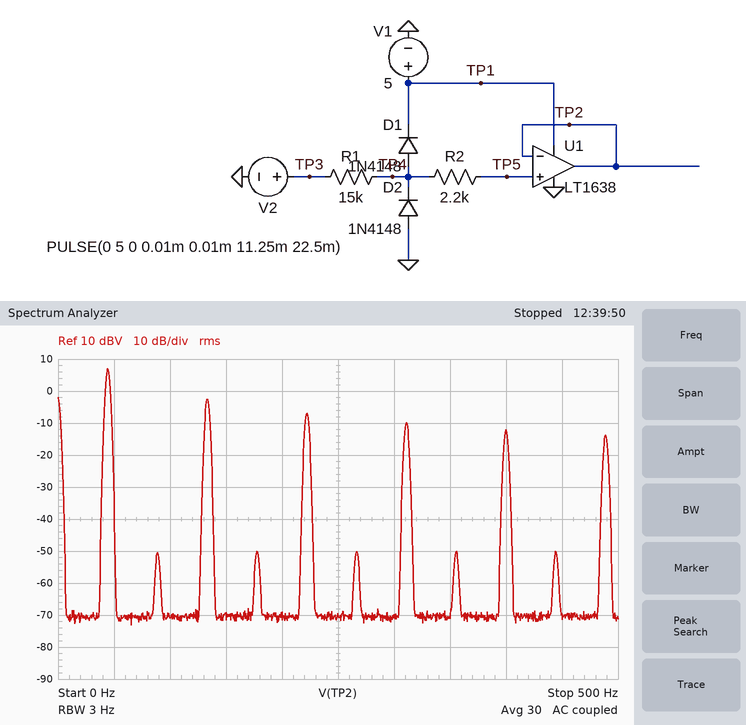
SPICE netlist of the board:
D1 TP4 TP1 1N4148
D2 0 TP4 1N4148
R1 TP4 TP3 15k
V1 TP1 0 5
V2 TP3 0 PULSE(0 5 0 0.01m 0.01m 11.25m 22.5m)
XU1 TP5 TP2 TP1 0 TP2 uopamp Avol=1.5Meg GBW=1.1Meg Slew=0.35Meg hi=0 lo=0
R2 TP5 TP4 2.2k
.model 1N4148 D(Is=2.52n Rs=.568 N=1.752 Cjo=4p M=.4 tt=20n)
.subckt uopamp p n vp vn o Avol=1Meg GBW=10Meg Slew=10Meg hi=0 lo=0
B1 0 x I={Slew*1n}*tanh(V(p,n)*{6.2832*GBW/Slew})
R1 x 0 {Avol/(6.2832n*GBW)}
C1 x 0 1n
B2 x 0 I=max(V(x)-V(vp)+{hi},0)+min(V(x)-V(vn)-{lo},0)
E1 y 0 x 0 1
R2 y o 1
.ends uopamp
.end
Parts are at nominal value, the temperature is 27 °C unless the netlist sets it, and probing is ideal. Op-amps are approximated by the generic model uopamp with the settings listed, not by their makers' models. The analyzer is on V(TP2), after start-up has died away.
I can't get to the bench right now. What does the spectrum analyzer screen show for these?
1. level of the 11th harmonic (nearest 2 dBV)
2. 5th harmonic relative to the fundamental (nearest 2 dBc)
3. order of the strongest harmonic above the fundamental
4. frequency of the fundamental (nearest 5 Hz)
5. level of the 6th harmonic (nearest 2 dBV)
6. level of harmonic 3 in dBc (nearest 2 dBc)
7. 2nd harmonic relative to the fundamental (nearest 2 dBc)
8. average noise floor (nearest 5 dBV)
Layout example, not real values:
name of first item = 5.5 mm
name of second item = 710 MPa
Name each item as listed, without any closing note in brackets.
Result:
level of the 11th harmonic = -14 dBV
5th harmonic relative to the fundamental = -14 dBc
order of the strongest harmonic above the fundamental = 3
frequency of the fundamental = 45 Hz
level of the 6th harmonic = -50 dBV
level of harmonic 3 in dBc = -10 dBc
2nd harmonic relative to the fundamental = -58 dBc
average noise floor = -70 dBV
